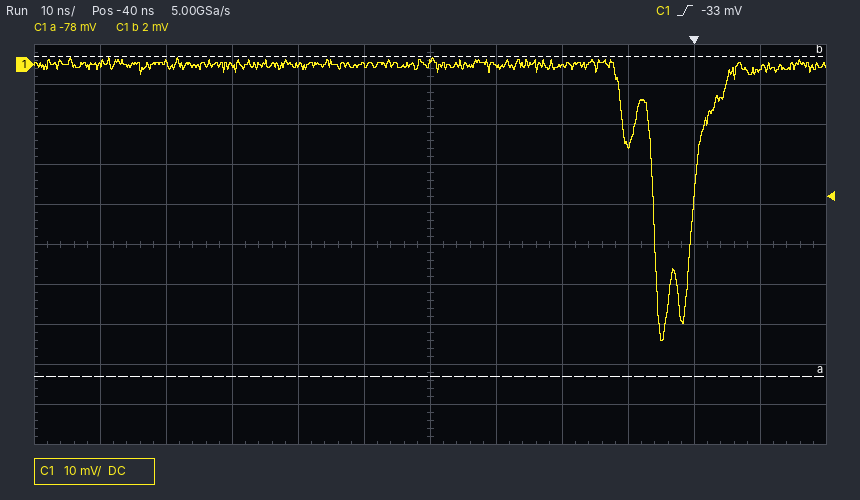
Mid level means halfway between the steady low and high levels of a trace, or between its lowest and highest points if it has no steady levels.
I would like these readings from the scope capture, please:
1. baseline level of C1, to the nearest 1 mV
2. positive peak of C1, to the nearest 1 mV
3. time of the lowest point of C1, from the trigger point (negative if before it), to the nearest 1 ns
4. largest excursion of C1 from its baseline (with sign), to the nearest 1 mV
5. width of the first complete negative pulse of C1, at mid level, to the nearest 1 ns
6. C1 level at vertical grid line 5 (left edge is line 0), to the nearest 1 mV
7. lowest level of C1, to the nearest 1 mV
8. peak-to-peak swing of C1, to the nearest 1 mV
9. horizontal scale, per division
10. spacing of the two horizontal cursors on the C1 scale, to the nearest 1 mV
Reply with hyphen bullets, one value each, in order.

- 0 mV
- 2 mV
- -5 ns
- -69 mV
- 6 ns
- 0 mV
- -69 mV
- 71 mV
- 10 ns
- 80 mV
